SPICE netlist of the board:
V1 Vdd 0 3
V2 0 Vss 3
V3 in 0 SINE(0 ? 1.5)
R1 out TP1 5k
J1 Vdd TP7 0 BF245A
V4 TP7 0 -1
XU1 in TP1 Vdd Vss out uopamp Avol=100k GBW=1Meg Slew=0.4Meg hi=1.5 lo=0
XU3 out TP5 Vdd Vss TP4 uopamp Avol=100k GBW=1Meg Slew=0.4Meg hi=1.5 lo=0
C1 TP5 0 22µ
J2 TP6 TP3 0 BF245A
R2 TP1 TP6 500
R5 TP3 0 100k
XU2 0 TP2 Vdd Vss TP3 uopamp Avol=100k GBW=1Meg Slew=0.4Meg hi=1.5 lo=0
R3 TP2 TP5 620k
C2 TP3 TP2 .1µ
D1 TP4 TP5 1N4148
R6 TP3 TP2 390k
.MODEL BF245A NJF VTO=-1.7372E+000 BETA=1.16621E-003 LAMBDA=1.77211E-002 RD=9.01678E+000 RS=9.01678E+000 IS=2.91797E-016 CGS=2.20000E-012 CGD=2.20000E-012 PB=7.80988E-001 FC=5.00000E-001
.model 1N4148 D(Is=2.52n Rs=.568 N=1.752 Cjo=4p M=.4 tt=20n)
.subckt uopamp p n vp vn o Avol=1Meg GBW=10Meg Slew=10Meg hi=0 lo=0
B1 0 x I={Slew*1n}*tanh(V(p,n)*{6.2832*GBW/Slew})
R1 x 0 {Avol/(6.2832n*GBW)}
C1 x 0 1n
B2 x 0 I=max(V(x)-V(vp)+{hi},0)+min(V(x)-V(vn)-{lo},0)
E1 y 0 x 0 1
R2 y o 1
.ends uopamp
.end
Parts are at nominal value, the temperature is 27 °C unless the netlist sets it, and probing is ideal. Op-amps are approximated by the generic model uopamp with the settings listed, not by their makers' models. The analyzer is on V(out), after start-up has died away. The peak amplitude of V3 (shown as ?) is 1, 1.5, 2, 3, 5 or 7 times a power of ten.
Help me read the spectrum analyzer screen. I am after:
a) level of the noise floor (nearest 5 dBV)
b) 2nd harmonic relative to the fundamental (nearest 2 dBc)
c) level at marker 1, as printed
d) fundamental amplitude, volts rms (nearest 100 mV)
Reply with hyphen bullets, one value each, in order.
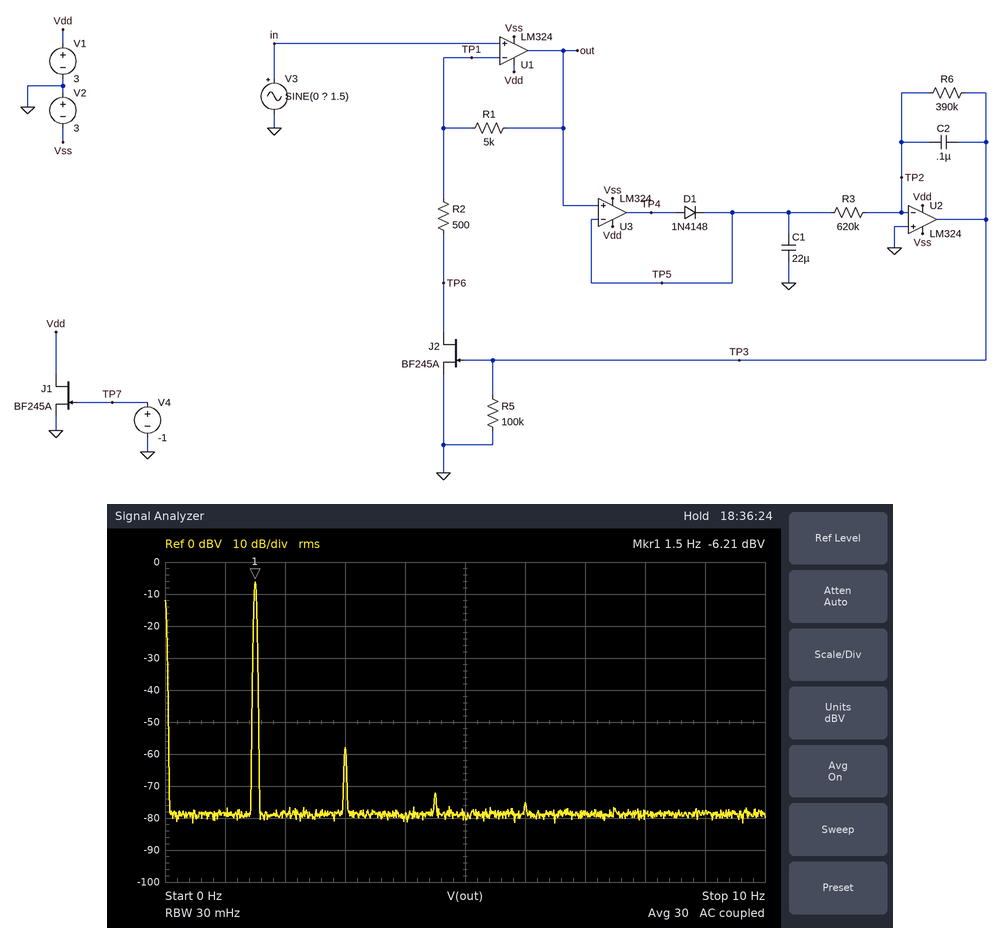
- -80 dBV
- -52 dBc
- -6.21 dBV
- 500 mV
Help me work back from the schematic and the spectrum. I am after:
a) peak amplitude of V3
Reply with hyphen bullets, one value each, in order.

- 100 mV
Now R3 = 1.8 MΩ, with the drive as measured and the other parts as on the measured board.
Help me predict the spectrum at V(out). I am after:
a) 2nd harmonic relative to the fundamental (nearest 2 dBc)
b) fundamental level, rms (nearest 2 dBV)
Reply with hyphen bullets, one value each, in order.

- -56 dBc
- -6 dBV
